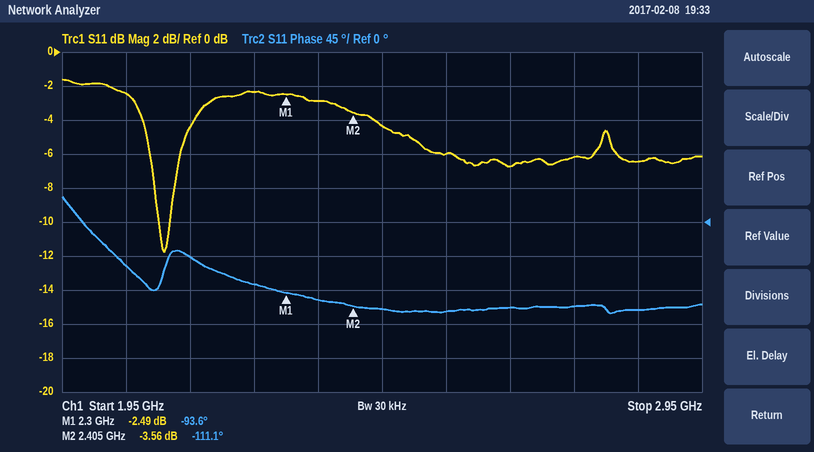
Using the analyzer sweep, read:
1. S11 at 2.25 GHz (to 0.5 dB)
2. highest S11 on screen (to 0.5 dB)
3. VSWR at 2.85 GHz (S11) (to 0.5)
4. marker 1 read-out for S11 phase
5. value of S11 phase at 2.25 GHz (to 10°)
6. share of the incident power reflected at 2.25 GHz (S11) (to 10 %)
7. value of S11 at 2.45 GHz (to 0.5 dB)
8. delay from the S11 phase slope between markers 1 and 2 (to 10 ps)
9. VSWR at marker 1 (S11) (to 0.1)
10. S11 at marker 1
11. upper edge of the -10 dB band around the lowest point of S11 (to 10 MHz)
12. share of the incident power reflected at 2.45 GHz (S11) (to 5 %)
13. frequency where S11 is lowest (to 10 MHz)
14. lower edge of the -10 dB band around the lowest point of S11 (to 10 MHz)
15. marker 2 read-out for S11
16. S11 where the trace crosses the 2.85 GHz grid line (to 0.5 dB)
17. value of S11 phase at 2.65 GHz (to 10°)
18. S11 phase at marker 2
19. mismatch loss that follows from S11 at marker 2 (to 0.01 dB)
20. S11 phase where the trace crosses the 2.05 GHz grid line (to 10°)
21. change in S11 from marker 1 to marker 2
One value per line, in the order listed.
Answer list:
-2.5 dB
-1.5 dB
3.0
-93.6°
-80°
60 %
-4.5 dB
460 ps
7.0
-2.49 dB
2.12 GHz
35 %
2.11 GHz
2.10 GHz
-3.56 dB
-6.5 dB
-110°
-111.1°
2.52 dB
-60°
-1.07 dB
